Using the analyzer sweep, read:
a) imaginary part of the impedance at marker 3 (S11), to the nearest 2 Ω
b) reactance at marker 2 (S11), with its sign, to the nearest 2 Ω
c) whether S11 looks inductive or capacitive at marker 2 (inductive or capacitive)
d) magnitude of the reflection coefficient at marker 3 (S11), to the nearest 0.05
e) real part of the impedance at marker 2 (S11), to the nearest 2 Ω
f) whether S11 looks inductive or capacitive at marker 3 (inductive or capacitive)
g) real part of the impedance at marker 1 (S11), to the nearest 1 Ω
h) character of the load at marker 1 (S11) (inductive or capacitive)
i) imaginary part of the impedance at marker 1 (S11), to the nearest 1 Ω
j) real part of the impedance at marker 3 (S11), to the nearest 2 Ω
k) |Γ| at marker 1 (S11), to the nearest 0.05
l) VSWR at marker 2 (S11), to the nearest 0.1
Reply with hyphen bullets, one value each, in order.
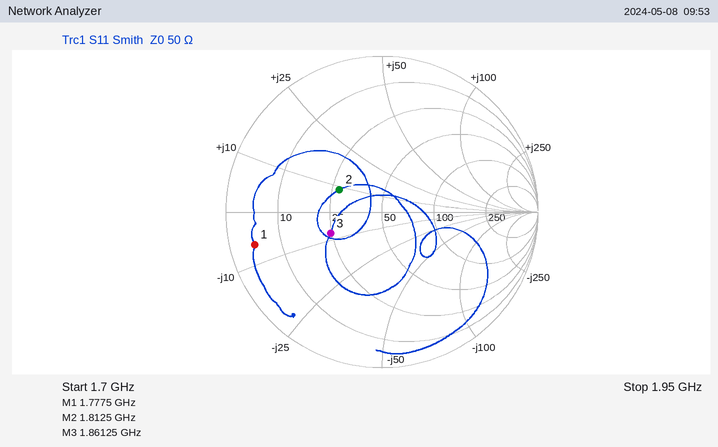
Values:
- -8 Ω
- +8 Ω
- inductive
- 0.35
- 28 Ω
- capacitive
- 4 Ω
- capacitive
- -6 Ω
- 24 Ω
- 0.85
- 1.9
